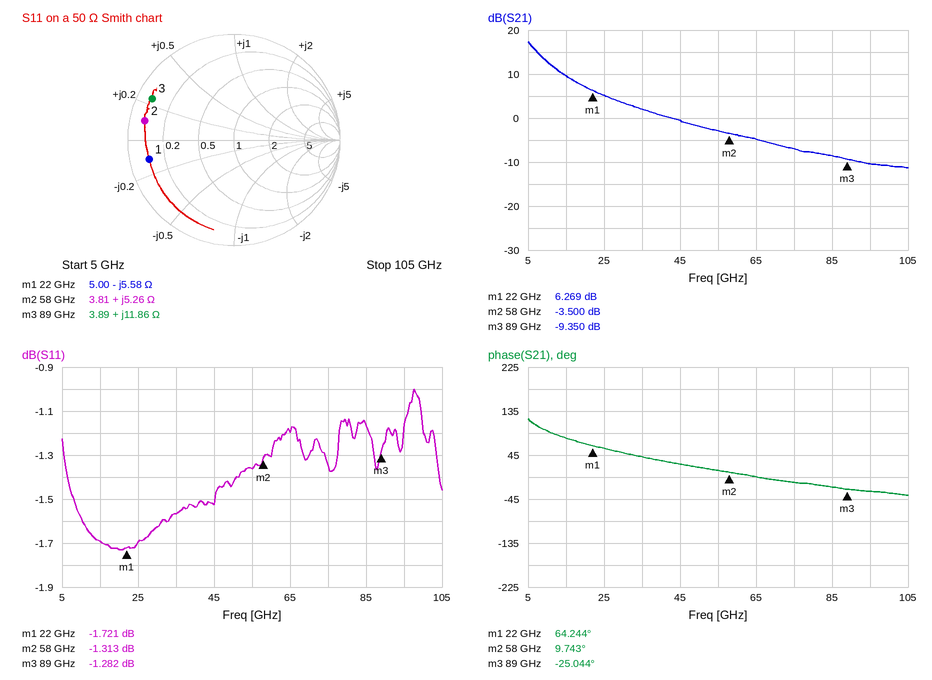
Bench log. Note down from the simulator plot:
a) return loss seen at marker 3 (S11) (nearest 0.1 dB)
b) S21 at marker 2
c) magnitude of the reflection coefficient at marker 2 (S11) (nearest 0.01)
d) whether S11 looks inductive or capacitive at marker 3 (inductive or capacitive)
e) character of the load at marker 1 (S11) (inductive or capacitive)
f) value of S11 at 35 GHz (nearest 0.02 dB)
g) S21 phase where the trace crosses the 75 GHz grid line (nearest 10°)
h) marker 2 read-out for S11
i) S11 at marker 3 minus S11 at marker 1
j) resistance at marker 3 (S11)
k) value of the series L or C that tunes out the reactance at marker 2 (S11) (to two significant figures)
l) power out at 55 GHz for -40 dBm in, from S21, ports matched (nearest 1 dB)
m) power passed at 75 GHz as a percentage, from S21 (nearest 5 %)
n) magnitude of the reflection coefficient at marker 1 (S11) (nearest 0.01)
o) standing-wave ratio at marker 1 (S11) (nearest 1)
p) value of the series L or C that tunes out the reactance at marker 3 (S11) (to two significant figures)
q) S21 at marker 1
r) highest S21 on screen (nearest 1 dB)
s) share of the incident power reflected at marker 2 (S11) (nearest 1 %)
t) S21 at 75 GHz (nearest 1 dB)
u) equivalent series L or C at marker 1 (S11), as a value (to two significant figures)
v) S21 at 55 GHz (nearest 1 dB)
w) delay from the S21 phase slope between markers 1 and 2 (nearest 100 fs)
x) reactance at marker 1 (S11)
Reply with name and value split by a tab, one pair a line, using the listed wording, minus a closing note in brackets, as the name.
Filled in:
return loss seen at marker 3 (S11)	1.3 dB
S21 at marker 2	-3.500 dB
magnitude of the reflection coefficient at marker 2 (S11)	0.86
whether S11 looks inductive or capacitive at marker 3	inductive
character of the load at marker 1 (S11)	capacitive
value of S11 at 35 GHz	-1.56 dB
S21 phase where the trace crosses the 75 GHz grid line	-10°
marker 2 read-out for S11	-1.313 dB
S11 at marker 3 minus S11 at marker 1	0.439 dB
resistance at marker 3	3.89 Ω
value of the series L or C that tunes out the reactance at marker 2 (S11)	520 fF
power out at 55 GHz for -40 dBm in, from S21, ports matched	-43 dBm
power passed at 75 GHz as a percentage, from S21	20 %
magnitude of the reflection coefficient at marker 1 (S11)	0.82
standing-wave ratio at marker 1 (S11)	10
value of the series L or C that tunes out the reactance at marker 3 (S11)	150 fF
S21 at marker 1	6.269 dB
highest S21 on screen	17 dB
share of the incident power reflected at marker 2 (S11)	74 %
S21 at 75 GHz	-7 dB
equivalent series L or C at marker 1 (S11), as a value	1.3 pF
S21 at 55 GHz	-3 dB
delay from the S21 phase slope between markers 1 and 2	4.2 ps
reactance at marker 1	-5.58 Ω
